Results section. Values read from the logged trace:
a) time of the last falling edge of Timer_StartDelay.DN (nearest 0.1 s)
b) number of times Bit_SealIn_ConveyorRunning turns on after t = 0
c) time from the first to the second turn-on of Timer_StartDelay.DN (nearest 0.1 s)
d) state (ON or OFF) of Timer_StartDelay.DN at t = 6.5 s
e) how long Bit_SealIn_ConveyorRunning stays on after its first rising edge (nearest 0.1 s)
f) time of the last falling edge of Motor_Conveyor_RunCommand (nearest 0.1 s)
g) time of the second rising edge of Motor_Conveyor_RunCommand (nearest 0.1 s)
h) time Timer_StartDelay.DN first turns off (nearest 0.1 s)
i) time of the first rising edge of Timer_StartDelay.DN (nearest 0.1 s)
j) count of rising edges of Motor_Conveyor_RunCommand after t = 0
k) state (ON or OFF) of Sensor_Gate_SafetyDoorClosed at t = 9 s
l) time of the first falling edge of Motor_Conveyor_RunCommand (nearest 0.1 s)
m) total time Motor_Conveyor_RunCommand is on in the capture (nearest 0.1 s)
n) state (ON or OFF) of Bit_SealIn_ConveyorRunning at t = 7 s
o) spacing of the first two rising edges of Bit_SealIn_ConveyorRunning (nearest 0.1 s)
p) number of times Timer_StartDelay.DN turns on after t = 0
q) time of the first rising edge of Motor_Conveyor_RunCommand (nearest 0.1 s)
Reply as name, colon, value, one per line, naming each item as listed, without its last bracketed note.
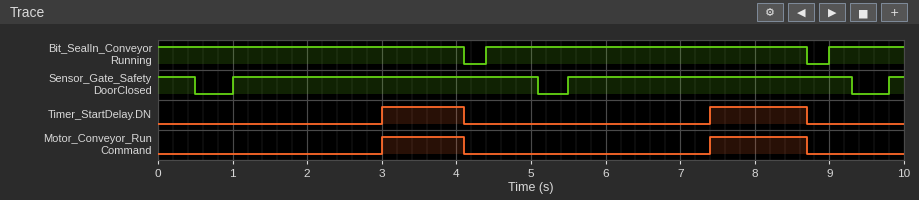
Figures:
time of the last falling edge of Timer_StartDelay.DN: 8.7 s
number of times Bit_SealIn_ConveyorRunning turns on after t = 0: 2
time from the first to the second turn-on of Timer_StartDelay.DN: 4.4 s
state (ON or OFF) of Timer_StartDelay.DN at t = 6.5 s: OFF
how long Bit_SealIn_ConveyorRunning stays on after its first rising edge: 4.3 s
time of the last falling edge of Motor_Conveyor_RunCommand: 8.7 s
time of the second rising edge of Motor_Conveyor_RunCommand: 7.4 s
time Timer_StartDelay.DN first turns off: 4.1 s
time of the first rising edge of Timer_StartDelay.DN: 3.0 s
count of rising edges of Motor_Conveyor_RunCommand after t = 0: 2
state (ON or OFF) of Sensor_Gate_SafetyDoorClosed at t = 9 s: ON
time of the first falling edge of Motor_Conveyor_RunCommand: 4.1 s
total time Motor_Conveyor_RunCommand is on in the capture: 2.4 s
state (ON or OFF) of Bit_SealIn_ConveyorRunning at t = 7 s: ON
spacing of the first two rising edges of Bit_SealIn_ConveyorRunning: 4.6 s
number of times Timer_StartDelay.DN turns on after t = 0: 2
time of the first rising edge of Motor_Conveyor_RunCommand: 3.0 s
